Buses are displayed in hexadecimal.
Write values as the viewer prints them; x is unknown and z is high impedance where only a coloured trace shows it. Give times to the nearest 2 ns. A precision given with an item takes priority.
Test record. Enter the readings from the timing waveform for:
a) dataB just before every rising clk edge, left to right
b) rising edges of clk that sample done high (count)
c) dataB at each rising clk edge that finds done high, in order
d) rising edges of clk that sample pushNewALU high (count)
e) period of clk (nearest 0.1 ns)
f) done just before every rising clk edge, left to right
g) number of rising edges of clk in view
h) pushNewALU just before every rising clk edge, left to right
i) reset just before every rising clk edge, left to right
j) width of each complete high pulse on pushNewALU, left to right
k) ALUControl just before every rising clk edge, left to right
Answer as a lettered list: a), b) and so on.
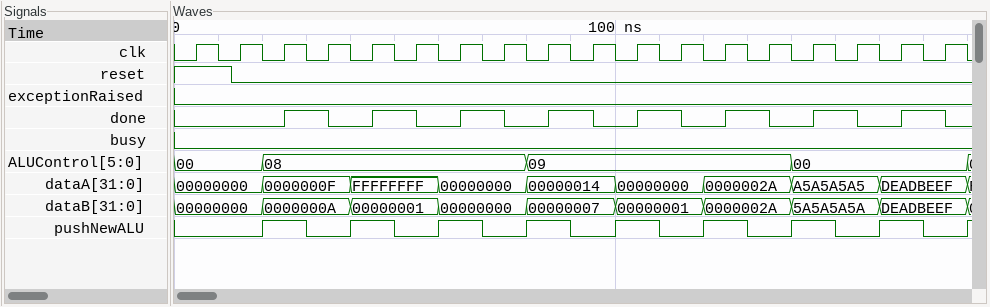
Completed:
a) 00000000, 00000000, 0000000A, 0000000A, 00000001, 00000001, 00000000, 00000000, 00000007, 00000007, 00000001, 00000001, 0000002A, 0000002A, 5A5A5A5A, 5A5A5A5A, DEADBEEF, DEADBEEF
b) 8
c) 0000000A, 00000001, 00000000, 00000007, 00000001, 0000002A, 5A5A5A5A, DEADBEEF
d) 8
e) 10 ns
f) 0 0 0 1 0 1 0 1 0 1 0 1 0 1 0 1 0 1
g) 18
h) 0 0 1 0 1 0 1 0 1 0 1 0 1 0 1 0 1 0
i) 1 0 0 0 0 0 0 0 0 0 0 0 0 0 0 0 0 0
j) 10 ns, 10 ns, 10 ns, 10 ns, 10 ns, 10 ns, 10 ns, 10 ns
k) 00, 00, 08, 08, 08, 08, 08, 08, 09, 09, 09, 09, 09, 09, 00, 00, 00, 00
